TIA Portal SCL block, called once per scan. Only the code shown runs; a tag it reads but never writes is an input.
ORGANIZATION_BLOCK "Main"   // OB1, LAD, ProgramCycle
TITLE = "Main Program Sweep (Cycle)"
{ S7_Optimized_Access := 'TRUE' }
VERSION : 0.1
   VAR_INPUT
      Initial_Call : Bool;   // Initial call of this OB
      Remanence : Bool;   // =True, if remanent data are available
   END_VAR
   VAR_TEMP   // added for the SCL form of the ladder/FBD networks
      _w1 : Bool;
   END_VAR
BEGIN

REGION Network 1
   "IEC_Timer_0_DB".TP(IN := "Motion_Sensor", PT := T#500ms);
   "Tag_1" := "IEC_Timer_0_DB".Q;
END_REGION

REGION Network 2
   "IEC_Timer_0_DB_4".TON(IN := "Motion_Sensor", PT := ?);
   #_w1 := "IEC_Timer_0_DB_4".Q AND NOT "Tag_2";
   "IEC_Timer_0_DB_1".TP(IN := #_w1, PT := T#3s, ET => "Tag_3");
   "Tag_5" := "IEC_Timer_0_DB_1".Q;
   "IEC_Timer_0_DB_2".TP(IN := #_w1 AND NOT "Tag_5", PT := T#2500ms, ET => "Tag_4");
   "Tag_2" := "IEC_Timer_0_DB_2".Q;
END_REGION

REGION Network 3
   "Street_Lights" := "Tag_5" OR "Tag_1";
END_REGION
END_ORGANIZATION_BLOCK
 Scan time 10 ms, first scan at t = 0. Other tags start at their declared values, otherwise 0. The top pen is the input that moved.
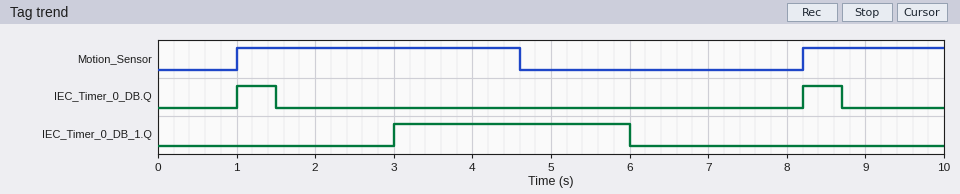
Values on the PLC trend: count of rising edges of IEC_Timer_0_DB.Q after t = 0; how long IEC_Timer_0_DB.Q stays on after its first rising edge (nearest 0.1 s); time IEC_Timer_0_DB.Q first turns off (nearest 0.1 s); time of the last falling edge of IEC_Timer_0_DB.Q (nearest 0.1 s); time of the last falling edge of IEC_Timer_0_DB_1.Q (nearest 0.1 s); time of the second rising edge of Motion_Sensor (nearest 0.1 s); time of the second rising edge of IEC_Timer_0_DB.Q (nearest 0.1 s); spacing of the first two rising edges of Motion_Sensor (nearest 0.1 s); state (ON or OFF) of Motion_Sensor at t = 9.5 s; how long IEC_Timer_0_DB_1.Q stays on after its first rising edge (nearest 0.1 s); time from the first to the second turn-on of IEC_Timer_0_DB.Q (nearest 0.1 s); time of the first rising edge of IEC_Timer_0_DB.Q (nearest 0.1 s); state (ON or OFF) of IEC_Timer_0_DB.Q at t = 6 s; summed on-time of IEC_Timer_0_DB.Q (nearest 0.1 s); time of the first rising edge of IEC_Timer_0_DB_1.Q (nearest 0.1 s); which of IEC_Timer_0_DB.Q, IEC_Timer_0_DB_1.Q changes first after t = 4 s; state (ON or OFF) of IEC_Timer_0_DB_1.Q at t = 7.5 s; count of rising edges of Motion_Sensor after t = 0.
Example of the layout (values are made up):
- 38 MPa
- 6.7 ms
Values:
- 2
- 0.5 s
- 1.5 s
- 8.7 s
- 6.0 s
- 8.2 s
- 8.2 s
- 7.2 s
- ON
- 3.0 s
- 7.2 s
- 1.0 s
- OFF
- 1.0 s
- 3.0 s
- IEC_Timer_0_DB_1.Q
- OFF
- 2
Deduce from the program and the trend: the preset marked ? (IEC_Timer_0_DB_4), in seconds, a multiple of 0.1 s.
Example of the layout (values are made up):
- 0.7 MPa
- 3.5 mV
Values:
- 2.0 s
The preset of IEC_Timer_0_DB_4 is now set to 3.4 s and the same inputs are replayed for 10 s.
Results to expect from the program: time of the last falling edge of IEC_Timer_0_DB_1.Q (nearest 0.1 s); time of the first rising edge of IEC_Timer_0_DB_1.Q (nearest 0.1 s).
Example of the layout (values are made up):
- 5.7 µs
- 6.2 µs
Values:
- 7.4 s
- 4.4 s
